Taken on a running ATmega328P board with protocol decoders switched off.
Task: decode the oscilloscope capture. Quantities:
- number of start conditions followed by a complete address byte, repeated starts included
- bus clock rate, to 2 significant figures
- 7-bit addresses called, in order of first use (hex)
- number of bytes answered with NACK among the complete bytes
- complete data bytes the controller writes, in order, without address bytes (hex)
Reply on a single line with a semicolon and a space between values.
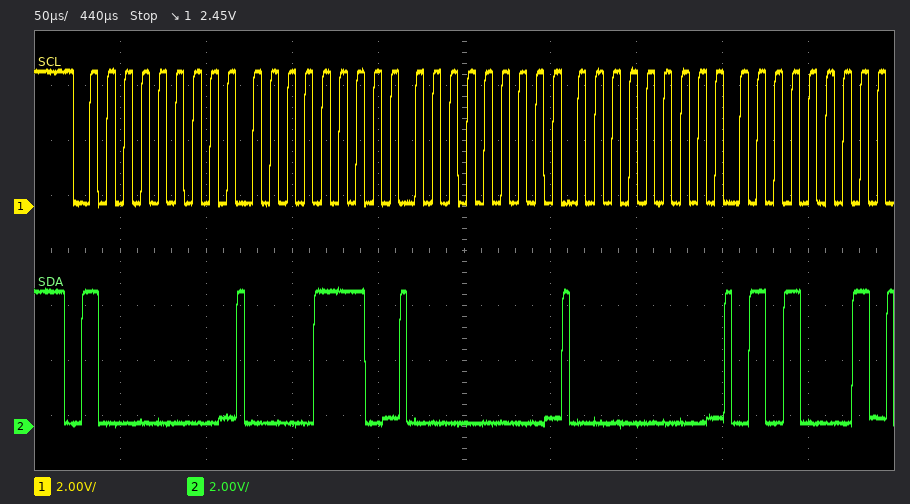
1; 100 kHz; 0x40; 0; 0E 00 00 51
